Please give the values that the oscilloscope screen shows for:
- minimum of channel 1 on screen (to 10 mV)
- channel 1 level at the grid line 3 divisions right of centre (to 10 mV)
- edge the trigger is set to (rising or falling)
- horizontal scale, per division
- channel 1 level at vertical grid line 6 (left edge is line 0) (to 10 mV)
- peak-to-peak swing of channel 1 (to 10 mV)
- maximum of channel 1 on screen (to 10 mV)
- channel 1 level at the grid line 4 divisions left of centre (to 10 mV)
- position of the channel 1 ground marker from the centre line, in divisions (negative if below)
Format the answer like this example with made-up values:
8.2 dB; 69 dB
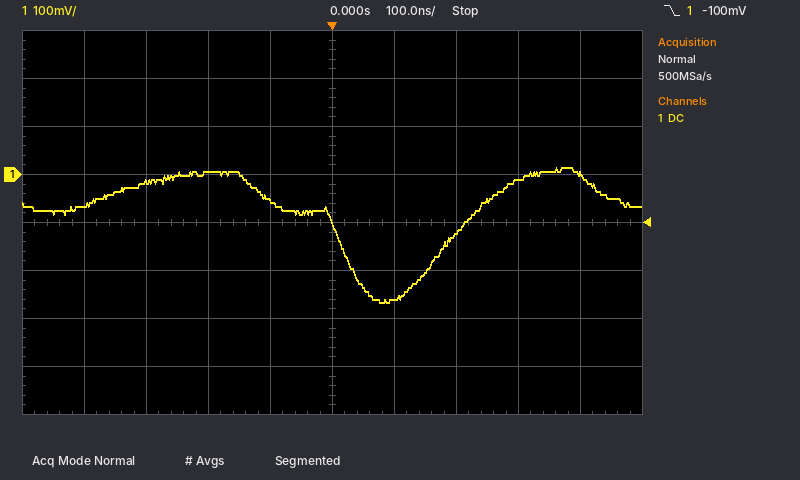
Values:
-270 mV; -10 mV; falling; 100 ns; -260 mV; 280 mV; 10 mV; -60 mV; +1.0 div
